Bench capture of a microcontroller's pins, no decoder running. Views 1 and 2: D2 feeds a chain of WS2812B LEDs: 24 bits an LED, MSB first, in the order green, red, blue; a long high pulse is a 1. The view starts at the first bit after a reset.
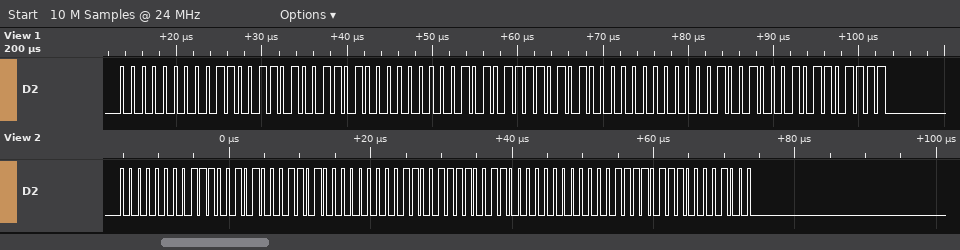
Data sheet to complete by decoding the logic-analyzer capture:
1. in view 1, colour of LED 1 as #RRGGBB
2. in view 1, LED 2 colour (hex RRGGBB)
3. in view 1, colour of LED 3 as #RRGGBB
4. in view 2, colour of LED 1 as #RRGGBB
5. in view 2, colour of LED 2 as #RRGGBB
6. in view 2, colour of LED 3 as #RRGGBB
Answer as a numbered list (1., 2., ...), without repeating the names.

1. #66009A
2. #AF0050
3. #91006F
4. #E5001A
5. #CF0030
6. #F70008
